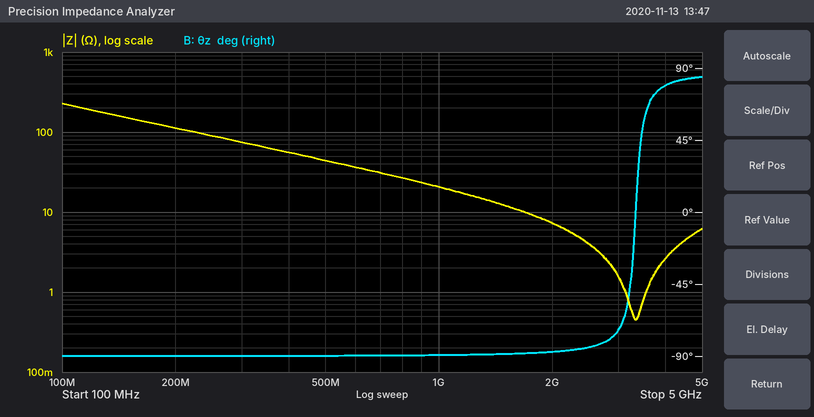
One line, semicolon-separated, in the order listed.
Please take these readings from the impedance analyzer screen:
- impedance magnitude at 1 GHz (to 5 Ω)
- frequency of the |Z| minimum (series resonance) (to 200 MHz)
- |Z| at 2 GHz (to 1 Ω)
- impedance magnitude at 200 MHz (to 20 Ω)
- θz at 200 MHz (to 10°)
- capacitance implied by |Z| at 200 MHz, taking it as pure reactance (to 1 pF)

20 Ω; 3.4 GHz; 7 Ω; 120 Ω; -90°; 7 pF
